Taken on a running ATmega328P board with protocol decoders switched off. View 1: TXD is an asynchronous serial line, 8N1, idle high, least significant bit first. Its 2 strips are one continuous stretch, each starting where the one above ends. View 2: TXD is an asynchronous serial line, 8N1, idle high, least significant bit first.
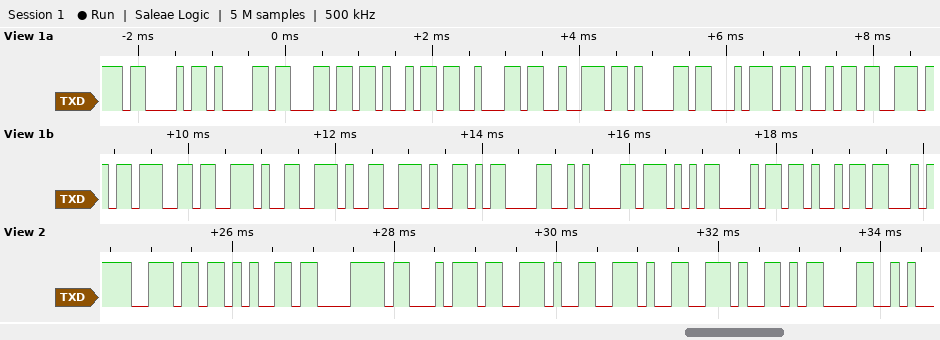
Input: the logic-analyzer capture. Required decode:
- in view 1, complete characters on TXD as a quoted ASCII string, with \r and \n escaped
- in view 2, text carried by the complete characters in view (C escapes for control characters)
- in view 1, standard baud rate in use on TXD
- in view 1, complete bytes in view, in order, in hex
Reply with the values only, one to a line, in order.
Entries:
"Calibrating...\r\nWhi"
"next...\r"
9600 baud
0x43 0x61 0x6C 0x69 0x62 0x72 0x61 0x74 0x69 0x6E 0x67 0x2E 0x2E 0x2E 0x0D 0x0A 0x57 0x68 0x69
